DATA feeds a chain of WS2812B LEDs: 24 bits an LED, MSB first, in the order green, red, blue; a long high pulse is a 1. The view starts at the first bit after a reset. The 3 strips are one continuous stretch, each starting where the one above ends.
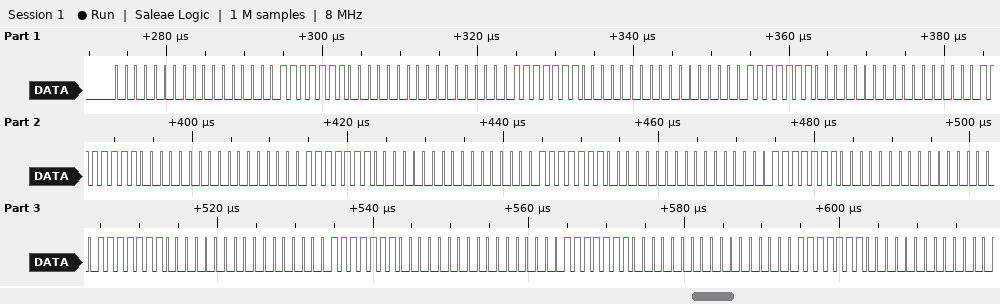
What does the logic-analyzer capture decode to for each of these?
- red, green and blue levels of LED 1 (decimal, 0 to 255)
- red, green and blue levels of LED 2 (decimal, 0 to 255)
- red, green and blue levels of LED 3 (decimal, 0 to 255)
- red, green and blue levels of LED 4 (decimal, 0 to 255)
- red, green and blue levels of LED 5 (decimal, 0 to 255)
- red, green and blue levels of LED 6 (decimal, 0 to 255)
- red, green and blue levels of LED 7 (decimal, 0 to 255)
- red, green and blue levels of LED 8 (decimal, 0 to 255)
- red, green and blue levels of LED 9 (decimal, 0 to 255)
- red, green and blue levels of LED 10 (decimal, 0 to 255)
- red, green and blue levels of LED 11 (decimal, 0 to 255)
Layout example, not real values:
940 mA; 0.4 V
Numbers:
0, 0, 127; 0, 0, 127; 0, 0, 127; 0, 0, 127; 0, 0, 127; 0, 0, 127; 0, 0, 127; 0, 0, 127; 0, 0, 127; 0, 0, 127; 0, 0, 127
